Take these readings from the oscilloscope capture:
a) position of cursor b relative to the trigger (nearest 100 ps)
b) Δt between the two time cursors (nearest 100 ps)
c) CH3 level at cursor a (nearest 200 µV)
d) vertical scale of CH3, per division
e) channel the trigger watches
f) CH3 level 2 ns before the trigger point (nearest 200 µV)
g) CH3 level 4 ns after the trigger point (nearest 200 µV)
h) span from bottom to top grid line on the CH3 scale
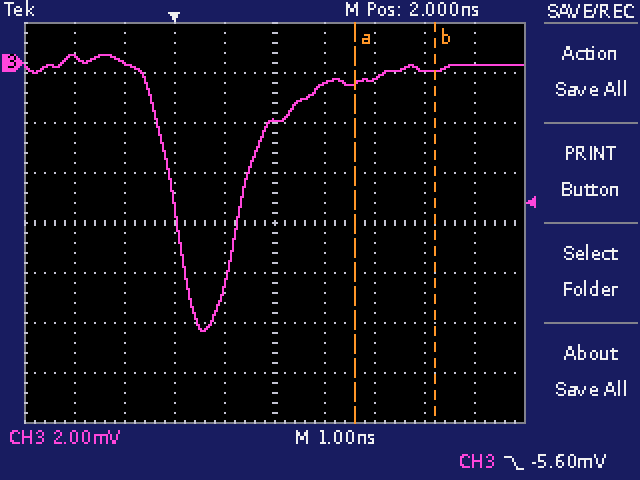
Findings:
+5.2 ns
1.6 ns
-800 µV
2 mV
CH3
200 µV
-600 µV
16 mV
